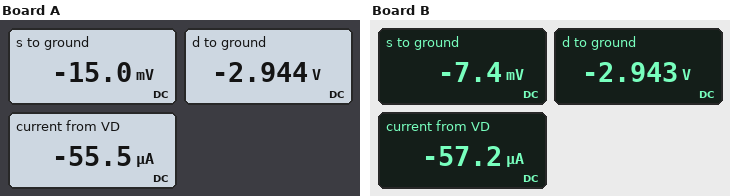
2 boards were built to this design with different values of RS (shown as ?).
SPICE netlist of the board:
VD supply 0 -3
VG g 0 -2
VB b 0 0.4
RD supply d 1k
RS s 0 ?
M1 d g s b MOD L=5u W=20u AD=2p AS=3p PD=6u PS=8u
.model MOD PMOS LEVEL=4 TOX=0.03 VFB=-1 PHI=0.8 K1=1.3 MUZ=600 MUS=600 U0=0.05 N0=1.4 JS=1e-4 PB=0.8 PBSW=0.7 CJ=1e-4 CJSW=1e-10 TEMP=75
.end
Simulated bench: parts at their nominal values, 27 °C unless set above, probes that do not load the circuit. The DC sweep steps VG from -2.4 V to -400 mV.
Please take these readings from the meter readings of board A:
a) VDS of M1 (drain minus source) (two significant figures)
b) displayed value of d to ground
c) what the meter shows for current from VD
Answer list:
-2.9 V
-2.944 V
-55.5 µA
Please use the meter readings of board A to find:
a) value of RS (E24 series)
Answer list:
270 Ω
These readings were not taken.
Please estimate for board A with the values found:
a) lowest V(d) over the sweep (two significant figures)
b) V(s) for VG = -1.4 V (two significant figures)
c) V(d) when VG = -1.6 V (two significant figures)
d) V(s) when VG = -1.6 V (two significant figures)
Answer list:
-3.0 V
-1.0 mV
-3.0 V
-3.9 mV
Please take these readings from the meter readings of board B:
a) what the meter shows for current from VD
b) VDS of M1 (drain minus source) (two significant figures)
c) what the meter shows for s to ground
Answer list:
-57.2 µA
-2.9 V
-7.4 mV
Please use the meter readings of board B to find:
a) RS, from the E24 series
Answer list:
130 Ω
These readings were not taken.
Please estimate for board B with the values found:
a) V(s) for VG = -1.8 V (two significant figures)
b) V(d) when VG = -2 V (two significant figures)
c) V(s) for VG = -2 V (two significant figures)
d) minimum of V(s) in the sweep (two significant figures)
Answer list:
-4.2 mV
-2.9 V
-7.4 mV
-16 mV
